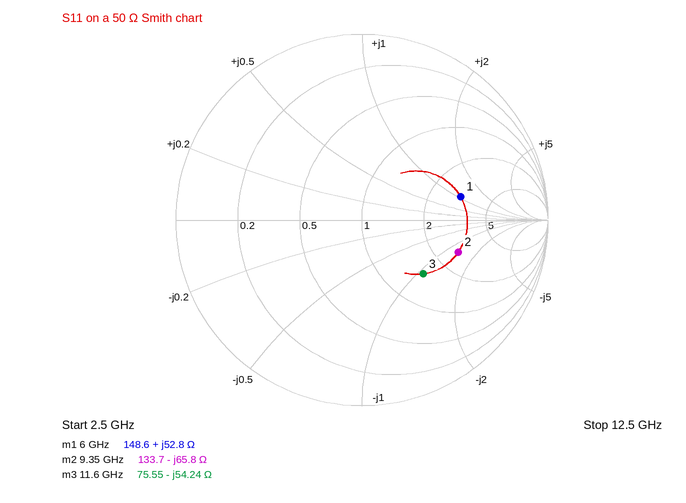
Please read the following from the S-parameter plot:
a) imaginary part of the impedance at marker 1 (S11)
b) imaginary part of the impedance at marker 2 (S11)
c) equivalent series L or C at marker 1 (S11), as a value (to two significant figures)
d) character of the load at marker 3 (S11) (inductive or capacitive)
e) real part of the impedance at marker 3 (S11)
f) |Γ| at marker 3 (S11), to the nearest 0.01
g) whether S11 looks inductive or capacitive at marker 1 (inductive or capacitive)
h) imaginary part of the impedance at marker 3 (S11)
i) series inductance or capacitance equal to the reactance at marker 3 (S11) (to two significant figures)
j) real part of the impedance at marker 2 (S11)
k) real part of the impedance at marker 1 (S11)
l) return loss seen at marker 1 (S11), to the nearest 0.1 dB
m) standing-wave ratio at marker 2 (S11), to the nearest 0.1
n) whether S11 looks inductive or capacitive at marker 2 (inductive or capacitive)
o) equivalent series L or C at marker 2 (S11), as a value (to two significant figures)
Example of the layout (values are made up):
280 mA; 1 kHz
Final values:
+52.8 Ω; -65.8 Ω; 1.4 nH; capacitive; 75.55 Ω; 0.44; inductive; -54.24 Ω; 250 fF; 133.7 Ω; 148.6 Ω; 5.3 dB; 3.4; capacitive; 260 fF
